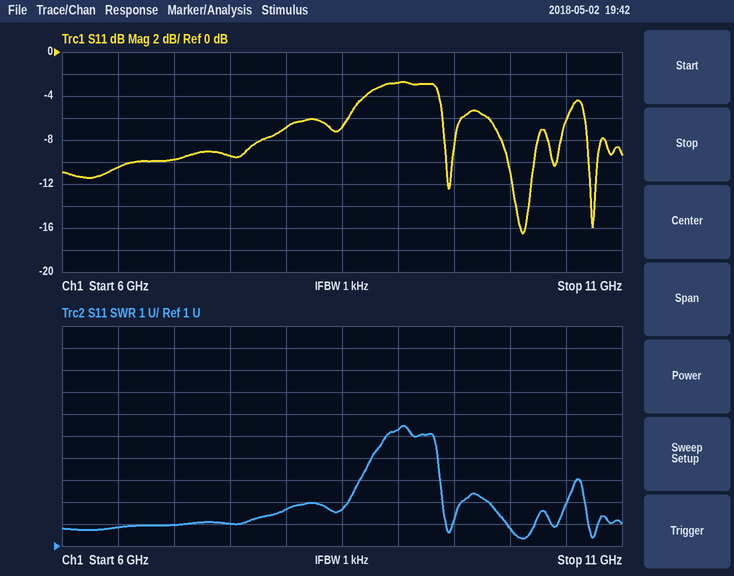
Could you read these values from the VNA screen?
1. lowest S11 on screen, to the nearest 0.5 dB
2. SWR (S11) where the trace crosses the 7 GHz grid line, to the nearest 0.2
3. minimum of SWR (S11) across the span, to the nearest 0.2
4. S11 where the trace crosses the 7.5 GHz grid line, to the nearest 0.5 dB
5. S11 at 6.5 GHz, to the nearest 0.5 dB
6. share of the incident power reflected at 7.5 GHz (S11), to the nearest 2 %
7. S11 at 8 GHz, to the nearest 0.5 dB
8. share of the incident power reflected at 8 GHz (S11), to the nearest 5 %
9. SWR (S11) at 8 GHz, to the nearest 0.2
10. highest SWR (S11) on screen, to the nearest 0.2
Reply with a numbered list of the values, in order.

1. -16.5 dB
2. 2.0
3. 1.4
4. -9.5 dB
5. -10.5 dB
6. 12 %
7. -7.0 dB
8. 20 %
9. 2.6
10. 6.4
